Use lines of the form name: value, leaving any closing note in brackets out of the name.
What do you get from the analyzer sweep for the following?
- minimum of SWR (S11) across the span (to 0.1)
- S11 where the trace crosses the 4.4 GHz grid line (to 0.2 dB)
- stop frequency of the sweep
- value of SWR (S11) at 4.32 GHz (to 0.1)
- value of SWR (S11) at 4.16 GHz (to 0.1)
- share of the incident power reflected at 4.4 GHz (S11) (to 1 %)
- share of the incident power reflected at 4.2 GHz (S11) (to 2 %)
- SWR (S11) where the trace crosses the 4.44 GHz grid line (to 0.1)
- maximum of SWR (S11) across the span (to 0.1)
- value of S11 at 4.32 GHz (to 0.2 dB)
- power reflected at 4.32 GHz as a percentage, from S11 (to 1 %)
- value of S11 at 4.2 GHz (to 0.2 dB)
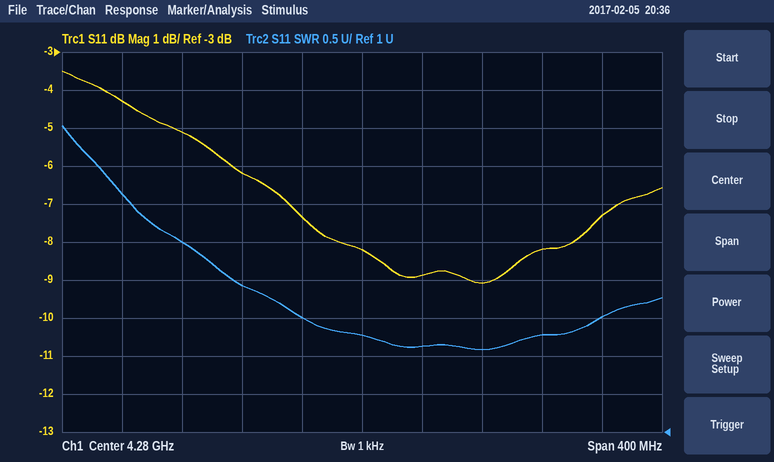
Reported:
minimum of SWR (S11) across the span: 2.1
S11 where the trace crosses the 4.4 GHz grid line: -8.2 dB
stop frequency of the sweep: 4.48 GHz
value of SWR (S11) at 4.32 GHz: 2.1
value of SWR (S11) at 4.16 GHz: 3.5
share of the incident power reflected at 4.4 GHz (S11): 15 %
share of the incident power reflected at 4.2 GHz (S11): 24 %
SWR (S11) where the trace crosses the 4.44 GHz grid line: 2.5
maximum of SWR (S11) across the span: 5.0
value of S11 at 4.32 GHz: -8.8 dB
power reflected at 4.32 GHz as a percentage, from S11: 13 %
value of S11 at 4.2 GHz: -6.2 dB
